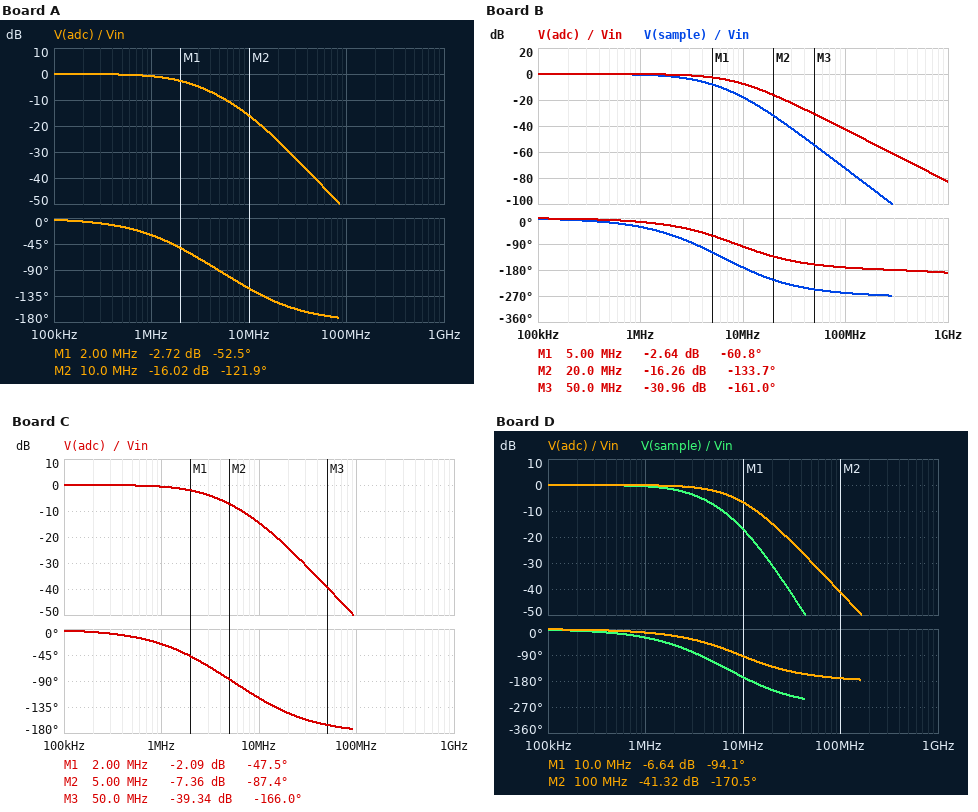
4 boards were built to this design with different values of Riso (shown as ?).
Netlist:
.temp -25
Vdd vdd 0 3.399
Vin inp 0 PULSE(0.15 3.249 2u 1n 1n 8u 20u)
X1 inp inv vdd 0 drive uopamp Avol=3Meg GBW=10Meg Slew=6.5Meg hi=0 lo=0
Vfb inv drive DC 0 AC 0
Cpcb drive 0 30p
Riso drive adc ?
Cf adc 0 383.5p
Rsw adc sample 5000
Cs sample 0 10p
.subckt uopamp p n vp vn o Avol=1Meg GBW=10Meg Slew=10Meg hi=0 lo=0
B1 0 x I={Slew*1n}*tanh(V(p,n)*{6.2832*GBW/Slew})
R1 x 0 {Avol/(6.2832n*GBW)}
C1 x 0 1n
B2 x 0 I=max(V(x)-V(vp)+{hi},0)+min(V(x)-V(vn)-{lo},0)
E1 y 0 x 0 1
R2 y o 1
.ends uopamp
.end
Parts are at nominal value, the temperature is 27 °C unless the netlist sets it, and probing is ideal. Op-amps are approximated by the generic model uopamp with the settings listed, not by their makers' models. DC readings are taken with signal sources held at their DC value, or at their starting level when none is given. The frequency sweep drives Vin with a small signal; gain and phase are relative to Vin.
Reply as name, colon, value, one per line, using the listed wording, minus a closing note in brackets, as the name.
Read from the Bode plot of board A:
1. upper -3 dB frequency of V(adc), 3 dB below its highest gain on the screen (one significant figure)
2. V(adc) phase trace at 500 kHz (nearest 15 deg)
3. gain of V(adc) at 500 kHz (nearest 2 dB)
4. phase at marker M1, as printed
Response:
upper -3 dB frequency of V(adc), 3 dB below its highest gain on the screen: 2 MHz
V(adc) phase trace at 500 kHz: -15 deg
gain of V(adc) at 500 kHz: 0 dB
phase at marker M1, as printed: -52.5 deg
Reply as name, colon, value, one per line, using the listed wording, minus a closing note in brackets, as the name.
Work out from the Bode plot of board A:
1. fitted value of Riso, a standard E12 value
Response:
fitted value of Riso, a standard E12 value: 180 Ω
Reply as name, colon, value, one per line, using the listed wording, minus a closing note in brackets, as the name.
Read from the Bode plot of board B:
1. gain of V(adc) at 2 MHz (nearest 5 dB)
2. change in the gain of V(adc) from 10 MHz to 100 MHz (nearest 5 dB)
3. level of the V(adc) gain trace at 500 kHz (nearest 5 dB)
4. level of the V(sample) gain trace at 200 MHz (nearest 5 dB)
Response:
gain of V(adc) at 2 MHz: 0 dB
change in the gain of V(adc) from 10 MHz to 100 MHz: -35 dB
level of the V(adc) gain trace at 500 kHz: 0 dB
level of the V(sample) gain trace at 200 MHz: -90 dB
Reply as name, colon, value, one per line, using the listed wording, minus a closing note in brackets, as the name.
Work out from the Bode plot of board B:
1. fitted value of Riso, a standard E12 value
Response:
fitted value of Riso, a standard E12 value: 56 Ω
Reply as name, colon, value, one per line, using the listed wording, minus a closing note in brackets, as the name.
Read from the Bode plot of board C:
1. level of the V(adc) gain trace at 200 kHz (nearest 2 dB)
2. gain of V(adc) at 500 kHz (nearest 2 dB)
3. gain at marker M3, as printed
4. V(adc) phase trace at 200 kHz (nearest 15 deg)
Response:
level of the V(adc) gain trace at 200 kHz: 0 dB
gain of V(adc) at 500 kHz: 0 dB
gain at marker M3, as printed: -39.34 dB
V(adc) phase trace at 200 kHz: 0 deg
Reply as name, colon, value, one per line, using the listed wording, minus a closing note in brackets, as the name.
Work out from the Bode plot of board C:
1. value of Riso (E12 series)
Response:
value of Riso: 150 Ω
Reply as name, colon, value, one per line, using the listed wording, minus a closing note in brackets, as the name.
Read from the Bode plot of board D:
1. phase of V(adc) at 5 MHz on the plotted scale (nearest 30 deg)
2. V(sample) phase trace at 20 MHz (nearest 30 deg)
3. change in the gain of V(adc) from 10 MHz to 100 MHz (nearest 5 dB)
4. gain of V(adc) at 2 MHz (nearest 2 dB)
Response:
phase of V(adc) at 5 MHz on the plotted scale: -60 deg
V(sample) phase trace at 20 MHz: -210 deg
change in the gain of V(adc) from 10 MHz to 100 MHz: -35 dB
gain of V(adc) at 2 MHz: 0 dB
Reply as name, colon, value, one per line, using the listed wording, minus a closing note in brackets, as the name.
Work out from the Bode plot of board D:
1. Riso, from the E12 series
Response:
Riso, from the E12 series: 47 Ω
